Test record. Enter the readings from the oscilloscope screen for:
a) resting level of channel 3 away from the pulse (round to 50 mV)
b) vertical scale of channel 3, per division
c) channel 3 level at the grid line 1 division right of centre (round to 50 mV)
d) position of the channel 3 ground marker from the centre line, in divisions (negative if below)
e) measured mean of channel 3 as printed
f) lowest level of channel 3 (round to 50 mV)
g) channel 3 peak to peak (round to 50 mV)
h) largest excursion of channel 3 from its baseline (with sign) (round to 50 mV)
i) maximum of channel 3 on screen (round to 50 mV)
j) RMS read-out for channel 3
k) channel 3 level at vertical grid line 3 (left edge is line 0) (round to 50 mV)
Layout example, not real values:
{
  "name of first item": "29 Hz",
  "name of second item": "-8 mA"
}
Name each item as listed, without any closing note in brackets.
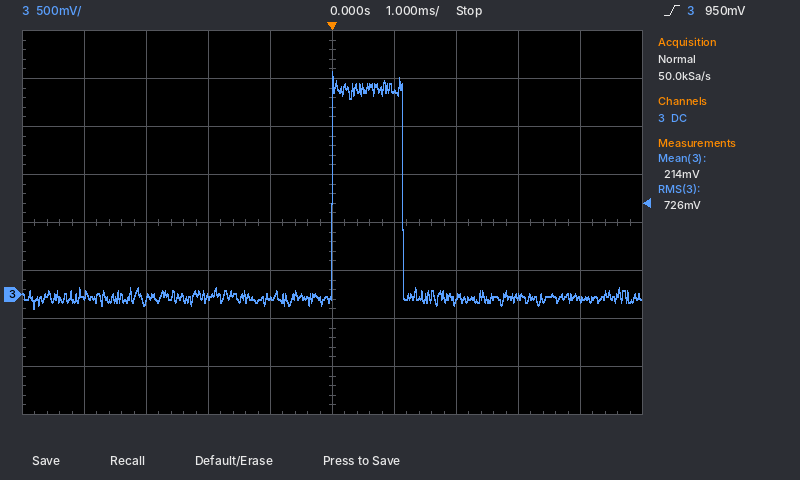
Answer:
{
  "resting level of channel 3 away from the pulse": "-50 mV",
  "vertical scale of channel 3, per division": "500 mV",
  "channel 3 level at the grid line 1 division right of centre": "2.15 V",
  "position of the channel 3 ground marker from the centre line, in divisions": "-1.5 div",
  "measured mean of channel 3 as printed": "214 mV",
  "lowest level of channel 3": "-150 mV",
  "channel 3 peak to peak": "2.45 V",
  "largest excursion of channel 3 from its baseline (with sign)": "+2.35 V",
  "maximum of channel 3 on screen": "2.30 V",
  "RMS read-out for channel 3": "726 mV",
  "channel 3 level at vertical grid line 3 (left edge is line 0)": "-50 mV"
}
